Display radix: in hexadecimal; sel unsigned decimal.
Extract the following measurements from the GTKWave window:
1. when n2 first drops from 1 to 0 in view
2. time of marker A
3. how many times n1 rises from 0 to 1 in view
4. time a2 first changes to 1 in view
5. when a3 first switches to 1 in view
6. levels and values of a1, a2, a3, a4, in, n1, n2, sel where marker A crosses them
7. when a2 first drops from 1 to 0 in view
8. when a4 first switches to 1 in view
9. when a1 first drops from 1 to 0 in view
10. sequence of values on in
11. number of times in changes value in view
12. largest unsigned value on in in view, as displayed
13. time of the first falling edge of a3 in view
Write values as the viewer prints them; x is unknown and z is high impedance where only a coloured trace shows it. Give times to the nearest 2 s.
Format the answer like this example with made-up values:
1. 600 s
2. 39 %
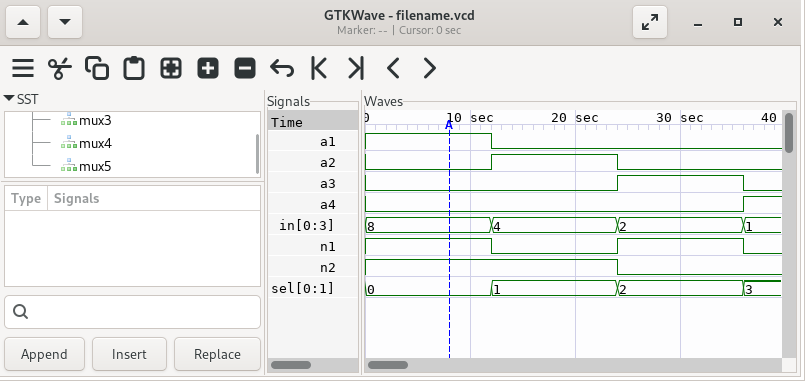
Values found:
1. 24 s
2. 8 s
3. 1
4. 12 s
5. 24 s
6. a1=1, a2=0, a3=0, a4=0, in=8, n1=1, n2=1, sel=0
7. 24 s
8. 36 s
9. 12 s
10. 8, 4, 2, 1
11. 3
12. 8
13. 36 s
